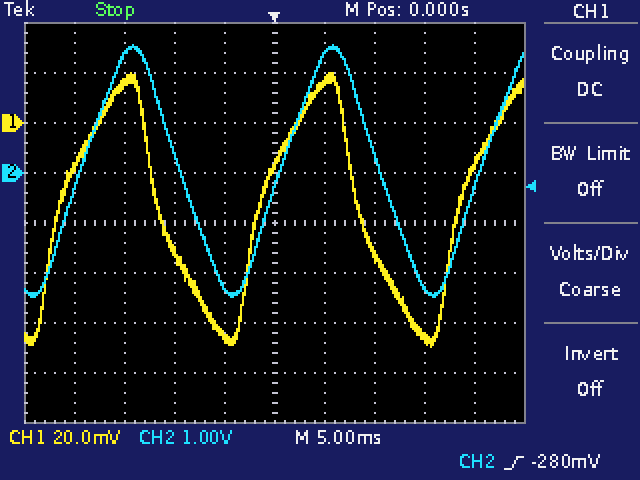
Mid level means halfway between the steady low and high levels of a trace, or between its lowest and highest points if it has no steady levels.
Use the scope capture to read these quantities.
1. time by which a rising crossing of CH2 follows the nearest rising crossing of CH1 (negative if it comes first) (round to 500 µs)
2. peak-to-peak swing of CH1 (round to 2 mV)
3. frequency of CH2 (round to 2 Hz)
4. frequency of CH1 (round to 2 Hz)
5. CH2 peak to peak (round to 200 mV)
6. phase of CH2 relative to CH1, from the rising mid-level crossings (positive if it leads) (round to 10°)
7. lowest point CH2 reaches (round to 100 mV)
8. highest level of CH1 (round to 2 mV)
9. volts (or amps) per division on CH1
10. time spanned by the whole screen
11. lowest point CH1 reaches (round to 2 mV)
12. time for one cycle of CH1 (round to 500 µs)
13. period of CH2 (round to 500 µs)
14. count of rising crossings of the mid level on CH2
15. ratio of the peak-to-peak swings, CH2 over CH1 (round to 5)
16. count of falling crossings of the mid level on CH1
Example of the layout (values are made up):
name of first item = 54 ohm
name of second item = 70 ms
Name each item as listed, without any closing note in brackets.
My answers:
time by which a rising crossing of CH2 follows the nearest rising crossing of CH1 (negative if it comes first) = +2.0 ms
peak-to-peak swing of CH1 = 110 mV
frequency of CH2 = 50 Hz
frequency of CH1 = 50 Hz
CH2 peak to peak = 5.0 V
phase of CH2 relative to CH1, from the rising mid-level crossings (positive if it leads) = -40°
lowest point CH2 reaches = -2.5 V
highest level of CH1 = 20 mV
volts (or amps) per division on CH1 = 20 mV
time spanned by the whole screen = 50 ms
lowest point CH1 reaches = -90 mV
time for one cycle of CH1 = 20.0 ms
period of CH2 = 20.0 ms
count of rising crossings of the mid level on CH2 = 3
ratio of the peak-to-peak swings, CH2 over CH1 = 45
count of falling crossings of the mid level on CH1 = 2
